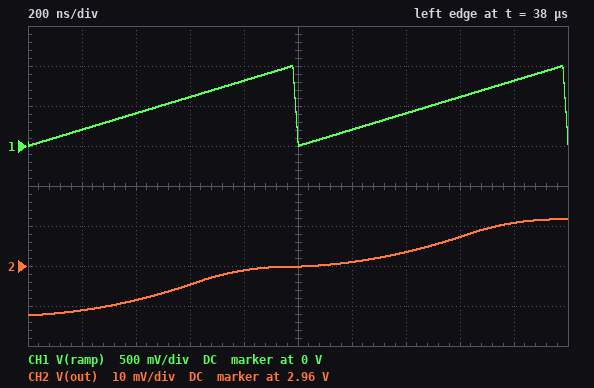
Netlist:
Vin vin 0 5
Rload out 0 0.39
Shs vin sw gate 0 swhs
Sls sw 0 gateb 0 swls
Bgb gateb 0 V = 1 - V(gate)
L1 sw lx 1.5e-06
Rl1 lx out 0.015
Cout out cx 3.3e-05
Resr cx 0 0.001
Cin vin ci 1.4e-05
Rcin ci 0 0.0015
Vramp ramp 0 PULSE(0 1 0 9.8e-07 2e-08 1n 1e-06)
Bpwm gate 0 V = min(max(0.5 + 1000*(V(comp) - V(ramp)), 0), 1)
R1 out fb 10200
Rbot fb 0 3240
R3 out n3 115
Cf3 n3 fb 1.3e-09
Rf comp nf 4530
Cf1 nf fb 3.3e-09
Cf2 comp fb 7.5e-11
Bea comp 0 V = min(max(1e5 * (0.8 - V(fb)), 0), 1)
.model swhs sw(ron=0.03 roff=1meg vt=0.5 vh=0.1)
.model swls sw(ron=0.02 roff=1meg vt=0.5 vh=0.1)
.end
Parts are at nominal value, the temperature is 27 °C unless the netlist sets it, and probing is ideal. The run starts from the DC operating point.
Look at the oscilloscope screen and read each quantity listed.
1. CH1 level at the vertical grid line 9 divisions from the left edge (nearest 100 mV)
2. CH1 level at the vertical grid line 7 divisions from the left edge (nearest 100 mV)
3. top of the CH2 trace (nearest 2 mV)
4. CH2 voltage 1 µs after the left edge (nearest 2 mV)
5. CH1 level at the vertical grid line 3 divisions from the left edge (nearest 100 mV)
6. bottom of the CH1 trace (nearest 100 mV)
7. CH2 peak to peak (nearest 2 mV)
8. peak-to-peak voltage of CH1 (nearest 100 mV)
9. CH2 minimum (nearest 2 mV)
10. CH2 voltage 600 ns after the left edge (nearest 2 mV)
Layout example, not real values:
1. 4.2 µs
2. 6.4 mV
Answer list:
1. 800 mV
2. 400 mV
3. 2.972 V
4. 2.960 V
5. 600 mV
6. 0 V
7. 24 mV
8. 1.0 V
9. 2.948 V
10. 2.956 V
